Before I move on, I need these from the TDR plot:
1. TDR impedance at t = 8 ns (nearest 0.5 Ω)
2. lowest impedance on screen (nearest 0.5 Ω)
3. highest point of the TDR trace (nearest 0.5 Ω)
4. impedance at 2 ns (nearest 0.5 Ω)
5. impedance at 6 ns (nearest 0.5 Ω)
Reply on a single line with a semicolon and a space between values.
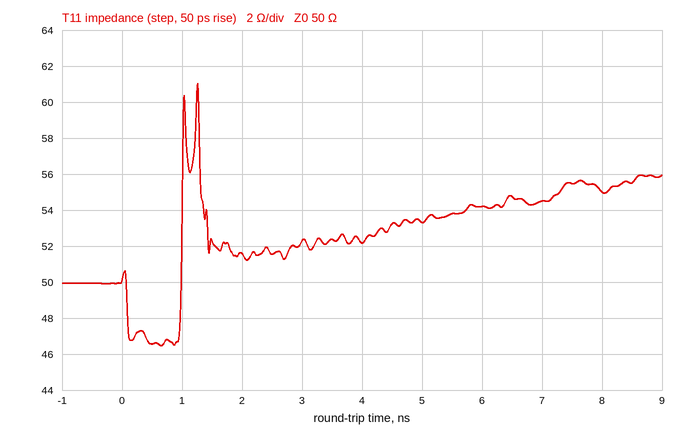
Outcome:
55.0 Ω; 46.5 Ω; 61.0 Ω; 51.5 Ω; 54.0 Ω
